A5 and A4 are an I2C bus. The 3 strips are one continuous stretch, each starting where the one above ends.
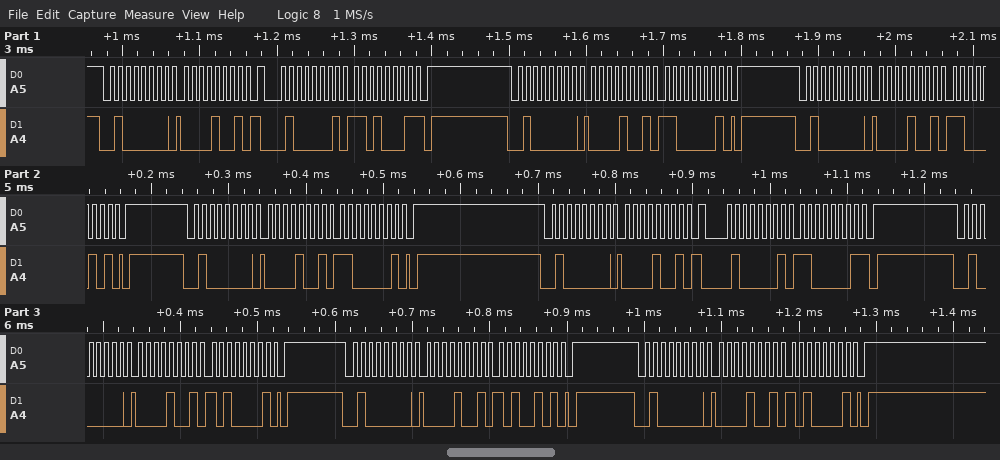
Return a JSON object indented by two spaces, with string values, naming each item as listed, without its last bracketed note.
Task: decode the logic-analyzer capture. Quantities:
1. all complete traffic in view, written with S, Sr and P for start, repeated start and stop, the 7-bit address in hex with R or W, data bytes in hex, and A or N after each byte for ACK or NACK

{
  "all complete traffic in view, written with S, Sr and P for start, repeated start and stop, the 7-bit address in hex with R or W, data bytes in hex, and A or N after each byte for ACK or NACK": "S 20W A 09 A Sr 20R A D1 N P S 20W A 09 A C1 A P S 20W A 09 A C5 A P S 20W A 09 A C1 A P S 20W A 09 A Sr 20R A C1 N P S 20W A 09 A A1 A P S 20W A 09 A A5 A P S 20W A 09 A A1 A P"
}
